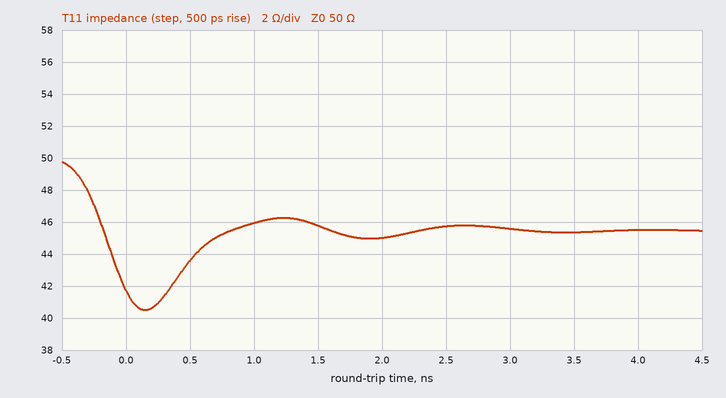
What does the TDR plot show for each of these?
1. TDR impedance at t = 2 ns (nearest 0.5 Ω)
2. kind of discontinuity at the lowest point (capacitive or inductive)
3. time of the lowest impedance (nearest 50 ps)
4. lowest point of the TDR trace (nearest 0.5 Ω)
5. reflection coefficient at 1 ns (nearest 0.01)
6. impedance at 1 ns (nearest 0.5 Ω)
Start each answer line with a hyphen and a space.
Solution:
- 45.0 Ω
- capacitive
- 150 ps
- 40.5 Ω
- -0.04
- 46.0 Ω
